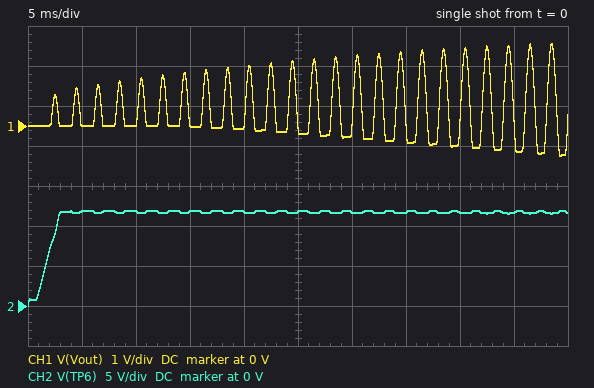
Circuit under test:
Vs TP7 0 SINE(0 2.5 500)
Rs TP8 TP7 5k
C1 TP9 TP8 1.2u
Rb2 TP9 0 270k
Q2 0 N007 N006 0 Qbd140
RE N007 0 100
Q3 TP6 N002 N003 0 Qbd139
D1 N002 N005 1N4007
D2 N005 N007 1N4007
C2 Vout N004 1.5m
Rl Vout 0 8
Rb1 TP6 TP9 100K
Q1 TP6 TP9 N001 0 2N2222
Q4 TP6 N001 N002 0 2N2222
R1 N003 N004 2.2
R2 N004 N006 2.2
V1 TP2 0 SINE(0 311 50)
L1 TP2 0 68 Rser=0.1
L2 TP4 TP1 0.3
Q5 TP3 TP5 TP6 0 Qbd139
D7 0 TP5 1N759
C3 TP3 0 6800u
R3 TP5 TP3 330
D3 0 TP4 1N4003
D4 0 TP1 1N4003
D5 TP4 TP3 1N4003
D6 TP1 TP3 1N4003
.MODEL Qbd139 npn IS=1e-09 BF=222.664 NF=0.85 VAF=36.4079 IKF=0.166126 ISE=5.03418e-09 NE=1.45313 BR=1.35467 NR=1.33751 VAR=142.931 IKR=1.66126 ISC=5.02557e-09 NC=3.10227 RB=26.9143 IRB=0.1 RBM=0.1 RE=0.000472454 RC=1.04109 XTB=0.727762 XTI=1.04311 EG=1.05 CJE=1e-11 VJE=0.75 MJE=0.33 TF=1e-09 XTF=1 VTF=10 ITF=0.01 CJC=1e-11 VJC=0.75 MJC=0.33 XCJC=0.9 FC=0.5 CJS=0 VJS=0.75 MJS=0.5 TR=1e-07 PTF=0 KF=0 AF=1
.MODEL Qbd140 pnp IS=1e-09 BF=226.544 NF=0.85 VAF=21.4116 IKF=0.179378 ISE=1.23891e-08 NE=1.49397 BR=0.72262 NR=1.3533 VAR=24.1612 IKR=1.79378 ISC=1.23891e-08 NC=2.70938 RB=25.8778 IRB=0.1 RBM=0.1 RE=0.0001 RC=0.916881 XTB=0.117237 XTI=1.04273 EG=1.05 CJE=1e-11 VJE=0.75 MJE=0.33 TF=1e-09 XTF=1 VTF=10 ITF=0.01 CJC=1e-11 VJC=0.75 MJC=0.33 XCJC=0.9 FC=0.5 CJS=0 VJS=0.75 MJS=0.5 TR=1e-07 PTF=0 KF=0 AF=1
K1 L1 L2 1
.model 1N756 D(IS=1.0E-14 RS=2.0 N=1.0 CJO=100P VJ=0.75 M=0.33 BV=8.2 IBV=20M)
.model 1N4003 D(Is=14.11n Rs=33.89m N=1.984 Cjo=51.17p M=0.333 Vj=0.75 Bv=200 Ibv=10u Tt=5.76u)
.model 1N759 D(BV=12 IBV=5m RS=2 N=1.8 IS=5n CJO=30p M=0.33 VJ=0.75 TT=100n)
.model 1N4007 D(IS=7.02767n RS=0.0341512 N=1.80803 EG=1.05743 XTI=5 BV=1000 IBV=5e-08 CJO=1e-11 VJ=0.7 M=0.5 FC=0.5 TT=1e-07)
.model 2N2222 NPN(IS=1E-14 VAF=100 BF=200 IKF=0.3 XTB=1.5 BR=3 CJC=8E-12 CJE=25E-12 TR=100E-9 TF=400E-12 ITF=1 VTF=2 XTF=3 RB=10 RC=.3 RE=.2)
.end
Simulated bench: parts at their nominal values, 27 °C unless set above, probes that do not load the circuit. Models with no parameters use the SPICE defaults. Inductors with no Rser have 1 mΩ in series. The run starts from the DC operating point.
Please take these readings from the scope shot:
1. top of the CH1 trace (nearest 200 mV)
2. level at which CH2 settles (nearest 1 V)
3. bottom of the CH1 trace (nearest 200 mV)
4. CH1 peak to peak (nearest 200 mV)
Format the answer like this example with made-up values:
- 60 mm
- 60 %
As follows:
- 2.0 V
- 12 V
- -800 mV
- 2.8 V
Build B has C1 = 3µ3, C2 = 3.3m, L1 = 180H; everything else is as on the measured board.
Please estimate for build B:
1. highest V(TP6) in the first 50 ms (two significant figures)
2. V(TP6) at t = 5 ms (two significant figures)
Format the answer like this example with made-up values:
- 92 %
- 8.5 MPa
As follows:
- 11 V
- 10 V
